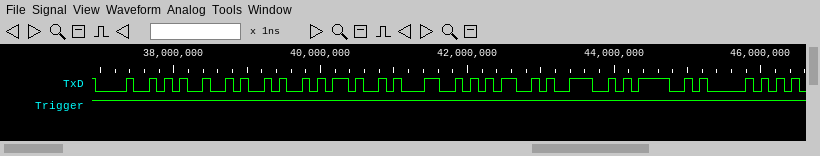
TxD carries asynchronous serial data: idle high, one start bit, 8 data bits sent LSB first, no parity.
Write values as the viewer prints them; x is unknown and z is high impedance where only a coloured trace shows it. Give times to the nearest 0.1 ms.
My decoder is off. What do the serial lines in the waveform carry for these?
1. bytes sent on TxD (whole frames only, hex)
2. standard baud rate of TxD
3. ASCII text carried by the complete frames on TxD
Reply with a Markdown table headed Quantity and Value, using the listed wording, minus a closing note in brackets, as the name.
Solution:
| Quantity | Value |
|---|---|
| bytes sent on TxD | 48, 49, 4A, 4B, 4C, 4D, 4E, 4F, 50 |
| standard baud rate of TxD | 9600 baud |
| ASCII text carried by the complete frames on TxD | "HIJKLMNOP" |
